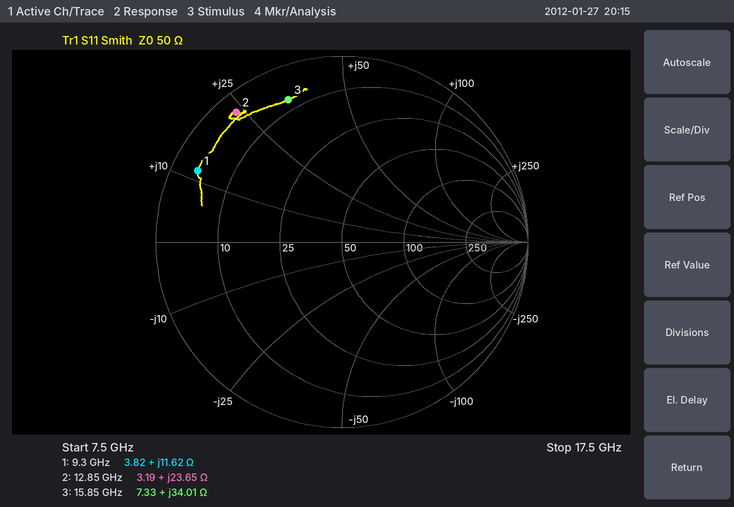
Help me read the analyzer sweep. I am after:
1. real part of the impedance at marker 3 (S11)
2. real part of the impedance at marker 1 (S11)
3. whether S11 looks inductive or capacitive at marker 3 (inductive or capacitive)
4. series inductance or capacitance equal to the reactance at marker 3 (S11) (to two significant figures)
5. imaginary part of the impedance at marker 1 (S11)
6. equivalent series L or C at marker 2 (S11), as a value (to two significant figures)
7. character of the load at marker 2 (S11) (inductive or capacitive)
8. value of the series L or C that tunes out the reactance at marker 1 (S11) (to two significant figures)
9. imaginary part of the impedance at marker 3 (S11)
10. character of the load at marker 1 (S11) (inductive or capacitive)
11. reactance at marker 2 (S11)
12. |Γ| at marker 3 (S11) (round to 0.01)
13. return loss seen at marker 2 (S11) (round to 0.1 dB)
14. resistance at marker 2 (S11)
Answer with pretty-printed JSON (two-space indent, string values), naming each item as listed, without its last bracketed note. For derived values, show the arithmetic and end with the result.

{
  "real part of the impedance at marker 3": "7.33 Ω",
  "real part of the impedance at marker 1": "3.82 Ω",
  "whether S11 looks inductive or capacitive at marker 3": "inductive",
  "series inductance or capacitance equal to the reactance at marker 3 (S11)": "L = 34.01 Ω/(2π × 15.85 GHz) ≈ 342 pH, so 340 pH to two significant figures",
  "imaginary part of the impedance at marker 1": "+11.62 Ω",
  "equivalent series L or C at marker 2 (S11), as a value": "L = 23.65 Ω/(2π × 12.85 GHz) ≈ 293 pH, so 290 pH to two significant figures",
  "character of the load at marker 2 (S11)": "inductive",
  "value of the series L or C that tunes out the reactance at marker 1 (S11)": "C = 1/(2π × 9.3 GHz × 11.62 Ω) ≈ 1.5 pF",
  "imaginary part of the impedance at marker 3": "+34.01 Ω",
  "character of the load at marker 1 (S11)": "inductive",
  "reactance at marker 2": "+23.65 Ω",
  "|Γ| at marker 3 (S11)": "0.82",
  "return loss seen at marker 2 (S11)": "0.9 dB",
  "resistance at marker 2": "3.19 Ω"
}
